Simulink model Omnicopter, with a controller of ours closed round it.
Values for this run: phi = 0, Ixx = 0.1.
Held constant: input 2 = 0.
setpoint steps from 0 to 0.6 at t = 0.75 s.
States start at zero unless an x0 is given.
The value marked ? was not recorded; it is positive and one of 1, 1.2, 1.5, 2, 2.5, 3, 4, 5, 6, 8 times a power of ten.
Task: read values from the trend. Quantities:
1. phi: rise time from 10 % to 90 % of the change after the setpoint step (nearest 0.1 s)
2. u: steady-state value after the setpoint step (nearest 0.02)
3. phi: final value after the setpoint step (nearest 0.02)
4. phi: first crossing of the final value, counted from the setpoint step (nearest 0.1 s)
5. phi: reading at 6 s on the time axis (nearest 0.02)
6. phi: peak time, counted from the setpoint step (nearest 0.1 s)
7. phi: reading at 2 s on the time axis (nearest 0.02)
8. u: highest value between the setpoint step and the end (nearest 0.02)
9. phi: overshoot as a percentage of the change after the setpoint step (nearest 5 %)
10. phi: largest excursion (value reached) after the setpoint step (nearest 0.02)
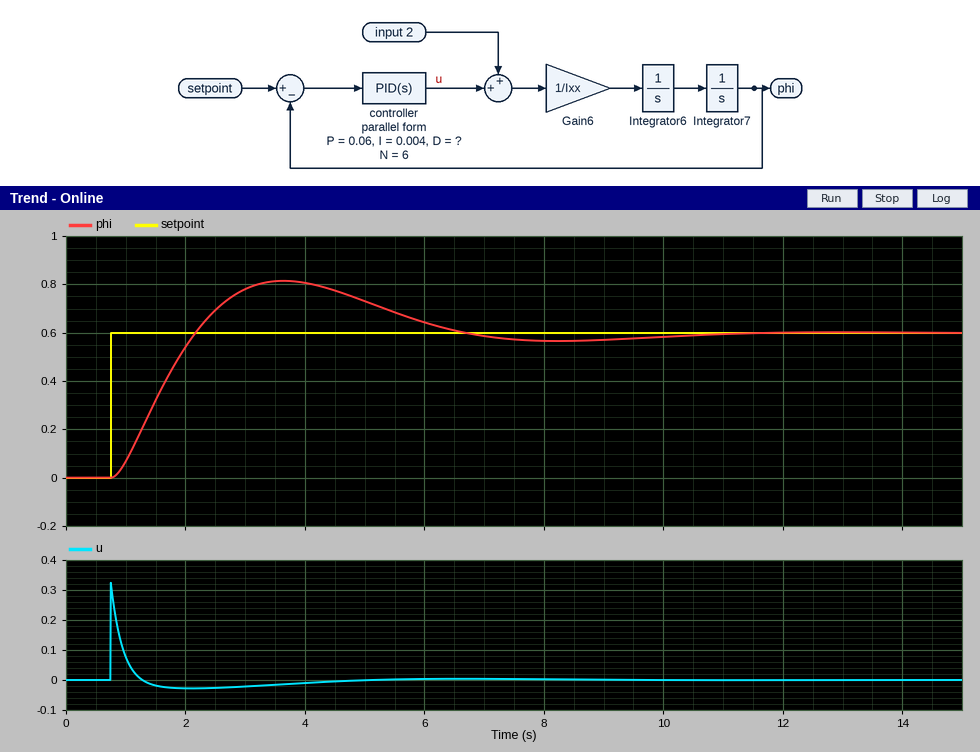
1.0 s
0.00
0.60
1.4 s
0.64
2.9 s
0.54
0.32
35 %
0.82
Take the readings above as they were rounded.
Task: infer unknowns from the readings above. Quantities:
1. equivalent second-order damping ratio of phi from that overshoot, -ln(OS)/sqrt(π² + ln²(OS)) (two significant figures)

0.32
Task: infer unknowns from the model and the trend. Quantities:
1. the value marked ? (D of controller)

0.08
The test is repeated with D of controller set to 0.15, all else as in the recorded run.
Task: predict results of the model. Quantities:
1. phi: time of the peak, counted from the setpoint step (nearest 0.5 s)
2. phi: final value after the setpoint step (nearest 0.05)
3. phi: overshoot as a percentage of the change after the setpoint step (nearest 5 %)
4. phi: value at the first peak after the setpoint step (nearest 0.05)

2.0 s
0.60
20 %
0.70
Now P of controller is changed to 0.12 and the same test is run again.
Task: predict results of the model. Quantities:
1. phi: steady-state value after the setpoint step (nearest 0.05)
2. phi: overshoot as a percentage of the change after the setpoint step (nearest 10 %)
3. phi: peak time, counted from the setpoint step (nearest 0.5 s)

0.60
50 %
2.0 s
